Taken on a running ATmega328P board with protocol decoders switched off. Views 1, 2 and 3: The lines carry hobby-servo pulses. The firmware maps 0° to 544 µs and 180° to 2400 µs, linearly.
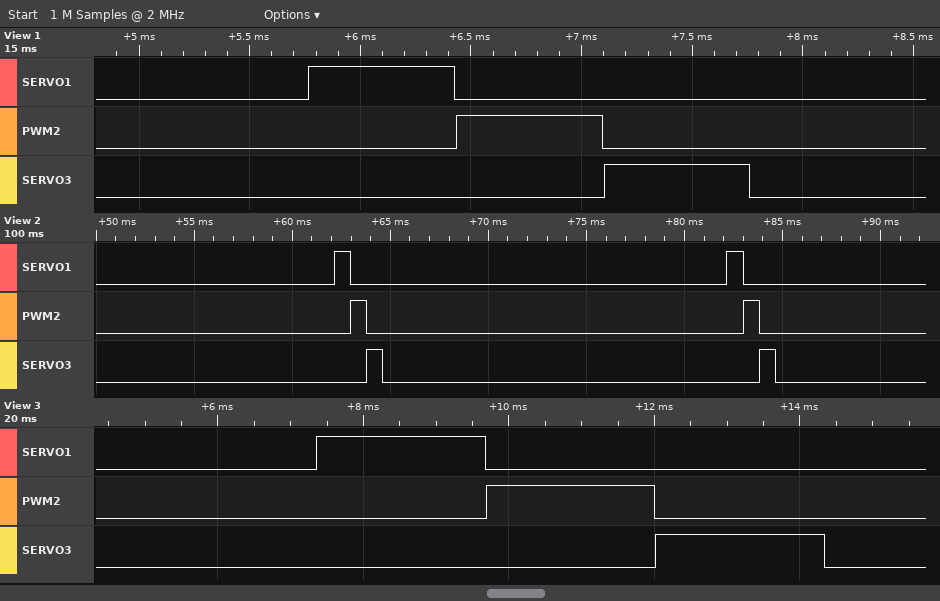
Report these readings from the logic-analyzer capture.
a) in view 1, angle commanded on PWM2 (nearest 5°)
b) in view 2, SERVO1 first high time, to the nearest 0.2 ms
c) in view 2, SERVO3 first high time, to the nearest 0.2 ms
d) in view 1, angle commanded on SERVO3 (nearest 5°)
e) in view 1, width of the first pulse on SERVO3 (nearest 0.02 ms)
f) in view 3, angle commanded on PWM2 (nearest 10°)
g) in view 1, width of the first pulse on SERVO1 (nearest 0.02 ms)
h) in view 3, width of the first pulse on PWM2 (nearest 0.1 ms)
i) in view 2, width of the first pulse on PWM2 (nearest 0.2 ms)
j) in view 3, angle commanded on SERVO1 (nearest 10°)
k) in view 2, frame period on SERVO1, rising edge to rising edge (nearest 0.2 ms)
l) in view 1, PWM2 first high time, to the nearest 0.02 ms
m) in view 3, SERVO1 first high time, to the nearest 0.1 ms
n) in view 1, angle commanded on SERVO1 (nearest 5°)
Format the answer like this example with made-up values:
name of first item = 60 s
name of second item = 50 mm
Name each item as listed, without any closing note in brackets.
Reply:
in view 1, angle commanded on PWM2 = 10°
in view 2, SERVO1 first high time, to the nearest 0.2 ms = 0.8 ms
in view 2, SERVO3 first high time, to the nearest 0.2 ms = 0.8 ms
in view 1, angle commanded on SERVO3 = 10°
in view 1, width of the first pulse on SERVO3 = 0.66 ms
in view 3, angle commanded on PWM2 = 170°
in view 1, width of the first pulse on SERVO1 = 0.66 ms
in view 3, width of the first pulse on PWM2 = 2.3 ms
in view 2, width of the first pulse on PWM2 = 0.8 ms
in view 3, angle commanded on SERVO1 = 170°
in view 2, frame period on SERVO1, rising edge to rising edge = 20.0 ms
in view 1, PWM2 first high time, to the nearest 0.02 ms = 0.66 ms
in view 3, SERVO1 first high time, to the nearest 0.1 ms = 2.3 ms
in view 1, angle commanded on SERVO1 = 10°
